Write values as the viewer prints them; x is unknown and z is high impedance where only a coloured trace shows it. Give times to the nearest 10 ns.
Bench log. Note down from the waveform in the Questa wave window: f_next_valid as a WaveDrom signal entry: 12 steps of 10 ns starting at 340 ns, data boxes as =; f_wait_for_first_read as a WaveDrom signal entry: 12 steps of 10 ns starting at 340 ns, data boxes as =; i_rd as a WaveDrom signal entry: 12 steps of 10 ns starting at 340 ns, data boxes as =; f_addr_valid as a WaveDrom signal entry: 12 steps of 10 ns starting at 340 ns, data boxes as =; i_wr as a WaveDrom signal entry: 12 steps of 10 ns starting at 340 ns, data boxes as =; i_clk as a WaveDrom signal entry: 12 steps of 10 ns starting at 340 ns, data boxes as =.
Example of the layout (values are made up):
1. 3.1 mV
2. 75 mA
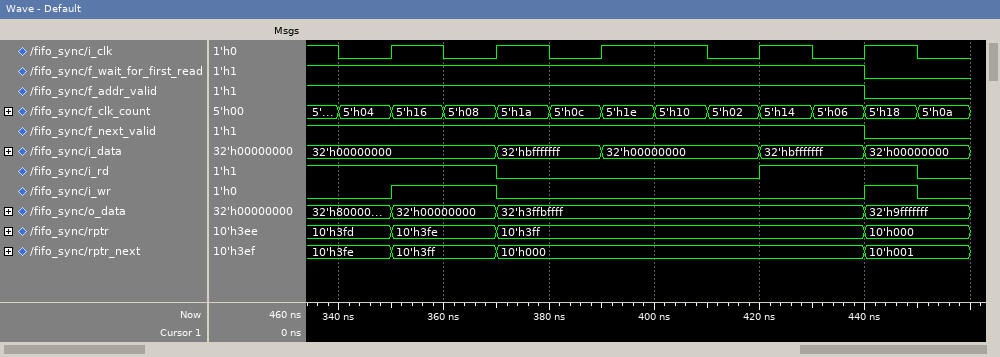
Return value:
1. {name: 'f_next_valid', wave: '1.........0.'}
2. {name: 'f_wait_for_first_read', wave: '1.........0.'}
3. {name: 'i_rd', wave: '1..0....1..0'}
4. {name: 'f_addr_valid', wave: '1.........0.'}
5. {name: 'i_wr', wave: '01.0......10'}
6. {name: 'i_clk', wave: '010101.01010'}
